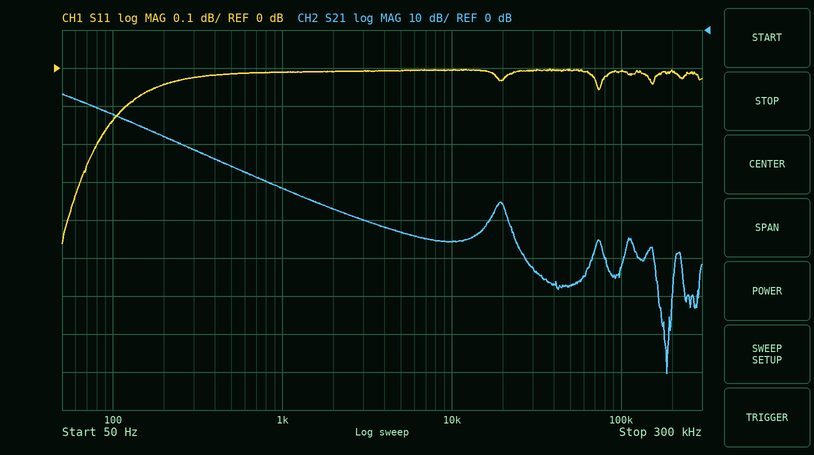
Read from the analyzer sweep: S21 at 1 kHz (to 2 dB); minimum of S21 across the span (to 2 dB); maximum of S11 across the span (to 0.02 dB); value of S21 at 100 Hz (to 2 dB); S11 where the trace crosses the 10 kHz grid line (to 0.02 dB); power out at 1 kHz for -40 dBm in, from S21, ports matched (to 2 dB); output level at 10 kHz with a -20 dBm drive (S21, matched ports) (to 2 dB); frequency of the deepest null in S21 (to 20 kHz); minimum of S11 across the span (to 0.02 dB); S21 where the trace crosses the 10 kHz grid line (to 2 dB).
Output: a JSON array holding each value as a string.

["-42 dB", "-90 dB", "0.00 dB", "-22 dB", "0.00 dB", "-82 dBm", "-76 dBm", "180 kHz", "-0.46 dB", "-56 dB"]
